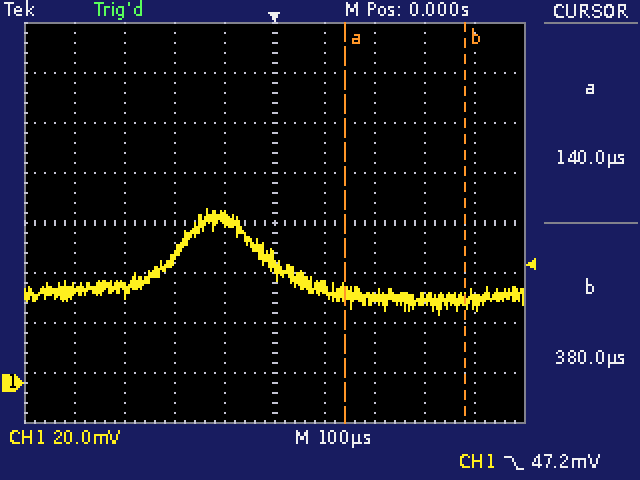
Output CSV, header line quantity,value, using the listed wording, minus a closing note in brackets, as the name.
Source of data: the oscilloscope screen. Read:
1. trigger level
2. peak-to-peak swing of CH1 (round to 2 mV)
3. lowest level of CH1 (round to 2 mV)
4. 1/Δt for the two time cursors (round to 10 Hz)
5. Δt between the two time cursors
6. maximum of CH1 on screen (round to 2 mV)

quantity,value
trigger level,47.2 mV
peak-to-peak swing of CH1,42 mV
lowest level of CH1,28 mV
1/Δt for the two time cursors,4.17 kHz
Δt between the two time cursors,240 µs
maximum of CH1 on screen,70 mV
